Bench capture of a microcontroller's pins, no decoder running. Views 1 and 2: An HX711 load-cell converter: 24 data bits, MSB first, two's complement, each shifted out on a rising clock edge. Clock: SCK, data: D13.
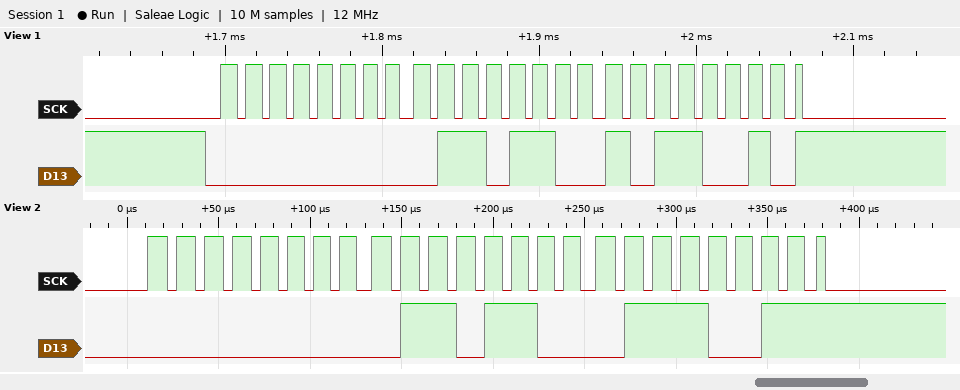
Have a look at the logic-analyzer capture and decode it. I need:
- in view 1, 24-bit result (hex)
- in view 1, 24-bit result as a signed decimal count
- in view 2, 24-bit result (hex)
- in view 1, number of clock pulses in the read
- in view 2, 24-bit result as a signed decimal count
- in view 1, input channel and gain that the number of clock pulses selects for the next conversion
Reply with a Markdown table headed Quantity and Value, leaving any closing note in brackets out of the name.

| Quantity | Value |
|---|---|
| in view 1, 24-bit result | 0x006CB2 |
| in view 1, 24-bit result as a signed decimal count | 27826 |
| in view 2, 24-bit result | 0x006C73 |
| in view 1, number of clock pulses in the read | 25 |
| in view 2, 24-bit result as a signed decimal count | 27763 |
| in view 1, input channel and gain that the number of clock pulses selects for the next conversion | channel A, gain 128 |
